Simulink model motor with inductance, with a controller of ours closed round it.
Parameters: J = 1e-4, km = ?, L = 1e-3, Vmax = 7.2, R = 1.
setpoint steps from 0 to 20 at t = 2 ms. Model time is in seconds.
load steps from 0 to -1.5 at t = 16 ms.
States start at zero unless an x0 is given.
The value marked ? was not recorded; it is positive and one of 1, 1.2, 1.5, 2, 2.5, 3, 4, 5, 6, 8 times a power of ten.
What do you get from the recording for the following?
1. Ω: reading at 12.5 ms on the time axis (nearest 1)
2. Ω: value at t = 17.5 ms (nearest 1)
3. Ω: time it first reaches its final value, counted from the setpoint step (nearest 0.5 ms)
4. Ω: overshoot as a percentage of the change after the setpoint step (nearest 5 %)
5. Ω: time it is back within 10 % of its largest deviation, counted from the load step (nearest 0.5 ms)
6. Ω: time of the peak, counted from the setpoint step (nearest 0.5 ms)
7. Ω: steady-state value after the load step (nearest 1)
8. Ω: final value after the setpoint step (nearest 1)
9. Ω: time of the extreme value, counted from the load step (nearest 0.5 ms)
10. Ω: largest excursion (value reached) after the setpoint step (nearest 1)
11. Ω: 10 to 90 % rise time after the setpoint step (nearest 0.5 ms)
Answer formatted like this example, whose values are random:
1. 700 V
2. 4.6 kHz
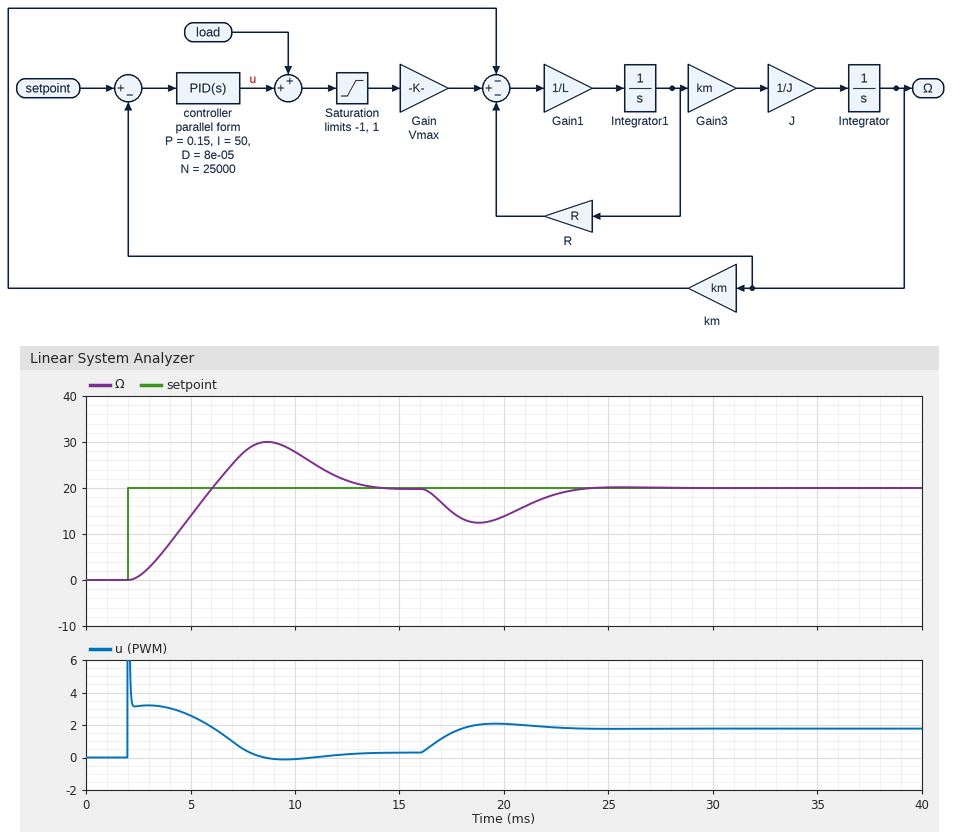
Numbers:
1. 22
2. 15
3. 4.0 ms
4. 50 %
5. 7.0 ms
6. 6.5 ms
7. 20
8. 20
9. 3.0 ms
10. 30
11. 3.0 ms
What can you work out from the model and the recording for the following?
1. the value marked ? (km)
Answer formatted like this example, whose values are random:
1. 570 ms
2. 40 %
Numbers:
1. 0.1
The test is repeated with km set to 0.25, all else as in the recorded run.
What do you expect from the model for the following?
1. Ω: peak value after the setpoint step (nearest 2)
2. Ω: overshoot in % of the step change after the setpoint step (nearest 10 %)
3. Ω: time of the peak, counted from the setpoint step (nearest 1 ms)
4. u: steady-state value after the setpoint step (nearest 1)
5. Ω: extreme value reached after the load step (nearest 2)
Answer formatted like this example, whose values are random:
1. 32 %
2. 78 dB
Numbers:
1. 24
2. 20 %
3. 3 ms
4. 1
5. 12
